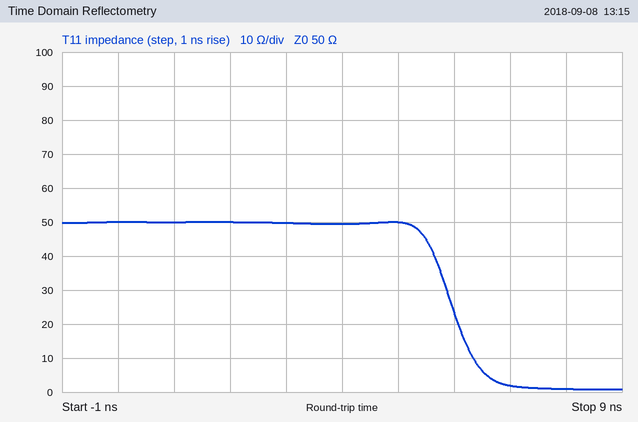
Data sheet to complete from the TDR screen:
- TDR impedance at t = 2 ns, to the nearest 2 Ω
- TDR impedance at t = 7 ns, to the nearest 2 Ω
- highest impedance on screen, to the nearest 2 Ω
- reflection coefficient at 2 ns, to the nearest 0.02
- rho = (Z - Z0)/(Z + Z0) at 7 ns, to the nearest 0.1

50 Ω
2 Ω
50 Ω
0.00
-0.9
